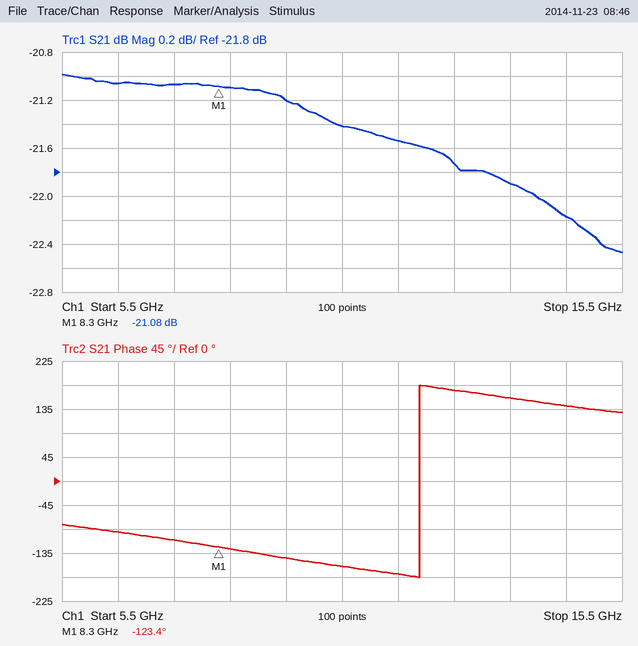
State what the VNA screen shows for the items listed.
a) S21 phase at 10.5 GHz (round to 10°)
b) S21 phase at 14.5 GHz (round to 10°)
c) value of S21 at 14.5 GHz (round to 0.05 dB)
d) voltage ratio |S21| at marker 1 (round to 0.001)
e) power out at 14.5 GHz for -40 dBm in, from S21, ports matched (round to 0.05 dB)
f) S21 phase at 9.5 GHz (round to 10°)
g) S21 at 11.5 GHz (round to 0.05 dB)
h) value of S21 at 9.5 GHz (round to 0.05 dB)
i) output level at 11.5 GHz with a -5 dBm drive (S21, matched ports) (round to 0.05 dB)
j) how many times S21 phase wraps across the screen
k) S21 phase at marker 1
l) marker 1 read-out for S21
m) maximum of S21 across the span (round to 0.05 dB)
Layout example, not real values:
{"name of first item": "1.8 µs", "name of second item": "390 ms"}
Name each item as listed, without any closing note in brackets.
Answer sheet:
{"S21 phase at 10.5 GHz": "-160°", "S21 phase at 14.5 GHz": "140°", "value of S21 at 14.5 GHz": "-22.15 dB", "voltage ratio |S21| at marker 1": "0.088", "power out at 14.5 GHz for -40 dBm in, from S21, ports matched": "-62.15 dBm", "S21 phase at 9.5 GHz": "-140°", "S21 at 11.5 GHz": "-21.55 dB", "value of S21 at 9.5 GHz": "-21.20 dB", "output level at 11.5 GHz with a -5 dBm drive (S21, matched ports)": "-26.55 dBm", "how many times S21 phase wraps across the screen": "1", "S21 phase at marker 1": "-123.4°", "marker 1 read-out for S21": "-21.08 dB", "maximum of S21 across the span": "-21.00 dB"}
